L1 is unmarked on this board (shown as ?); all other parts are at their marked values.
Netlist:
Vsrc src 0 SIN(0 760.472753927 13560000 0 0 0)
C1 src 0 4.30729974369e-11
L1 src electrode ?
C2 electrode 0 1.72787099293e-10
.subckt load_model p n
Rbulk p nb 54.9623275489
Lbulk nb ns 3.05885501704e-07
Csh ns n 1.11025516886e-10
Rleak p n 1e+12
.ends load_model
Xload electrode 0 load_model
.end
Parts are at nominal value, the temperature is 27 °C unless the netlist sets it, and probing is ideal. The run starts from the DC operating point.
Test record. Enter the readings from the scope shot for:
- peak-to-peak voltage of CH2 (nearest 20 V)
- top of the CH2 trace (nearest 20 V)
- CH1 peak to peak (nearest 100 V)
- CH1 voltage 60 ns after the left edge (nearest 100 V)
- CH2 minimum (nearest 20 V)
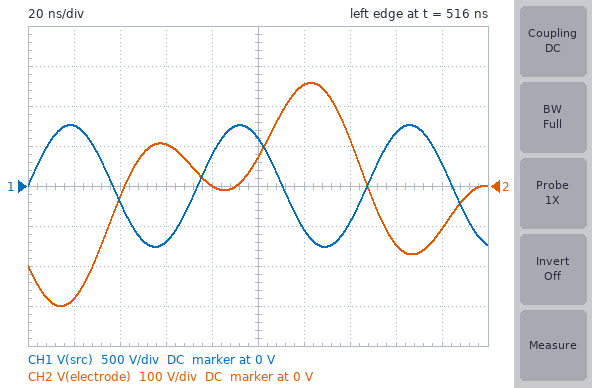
560 V
260 V
1.5 kV
-700 V
-300 V
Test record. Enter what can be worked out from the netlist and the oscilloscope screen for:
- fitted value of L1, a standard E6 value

3.3 µH
